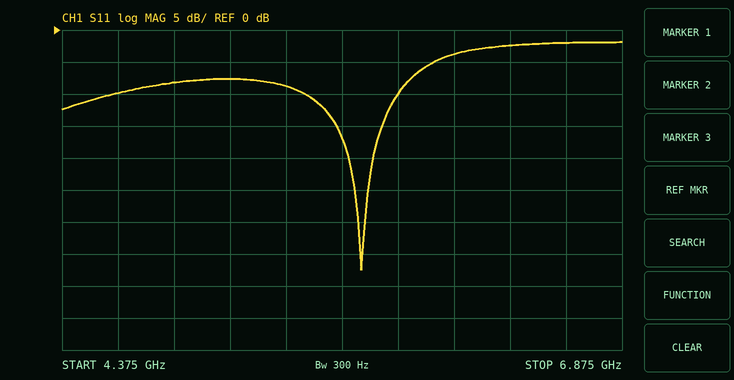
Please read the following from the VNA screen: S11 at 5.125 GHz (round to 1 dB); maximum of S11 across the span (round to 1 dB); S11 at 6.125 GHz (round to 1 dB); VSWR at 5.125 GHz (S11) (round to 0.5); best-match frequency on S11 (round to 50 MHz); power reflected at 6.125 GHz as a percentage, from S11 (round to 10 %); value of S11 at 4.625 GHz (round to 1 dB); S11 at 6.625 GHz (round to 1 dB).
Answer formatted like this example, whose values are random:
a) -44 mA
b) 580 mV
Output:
a) -8 dB
b) -2 dB
c) -4 dB
d) 2.5
e) 5.70 GHz
f) 40 %
g) -10 dB
h) -2 dB
